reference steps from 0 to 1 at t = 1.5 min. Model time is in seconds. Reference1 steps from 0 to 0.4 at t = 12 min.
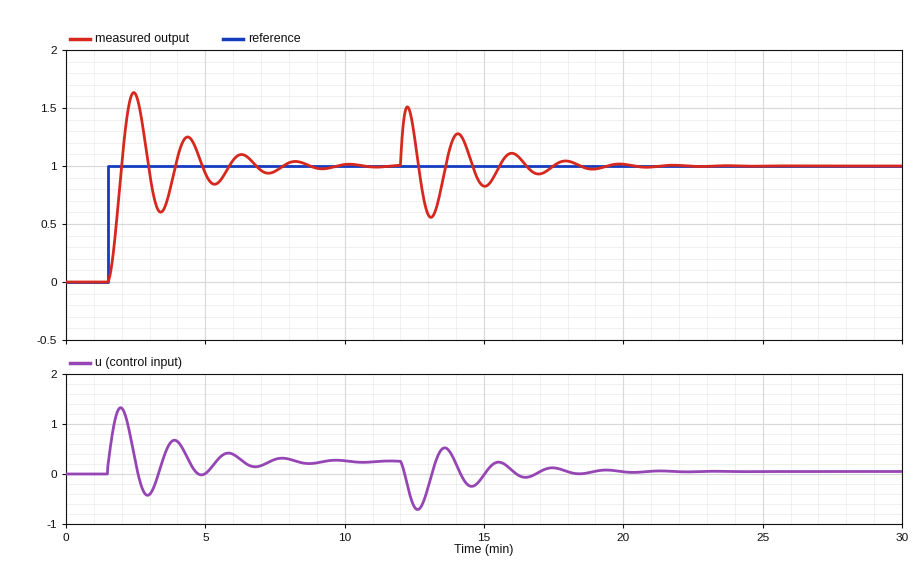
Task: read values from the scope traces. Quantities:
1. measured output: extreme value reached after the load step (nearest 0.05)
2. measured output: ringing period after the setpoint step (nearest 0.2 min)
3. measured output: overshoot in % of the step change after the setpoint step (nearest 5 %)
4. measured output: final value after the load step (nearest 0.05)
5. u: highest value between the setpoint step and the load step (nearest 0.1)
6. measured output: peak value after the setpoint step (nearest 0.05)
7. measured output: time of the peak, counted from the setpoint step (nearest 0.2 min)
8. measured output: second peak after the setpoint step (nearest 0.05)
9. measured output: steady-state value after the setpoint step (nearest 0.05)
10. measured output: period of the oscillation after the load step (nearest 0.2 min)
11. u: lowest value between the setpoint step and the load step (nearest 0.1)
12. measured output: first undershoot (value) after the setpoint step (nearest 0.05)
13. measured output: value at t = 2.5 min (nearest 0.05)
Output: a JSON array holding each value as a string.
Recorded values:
["1.50", "2.0 min", "65 %", "1.00", "1.3", "1.65", "1.0 min", "1.25", "1.00", "1.8 min", "-0.4", "0.60", "1.60"]
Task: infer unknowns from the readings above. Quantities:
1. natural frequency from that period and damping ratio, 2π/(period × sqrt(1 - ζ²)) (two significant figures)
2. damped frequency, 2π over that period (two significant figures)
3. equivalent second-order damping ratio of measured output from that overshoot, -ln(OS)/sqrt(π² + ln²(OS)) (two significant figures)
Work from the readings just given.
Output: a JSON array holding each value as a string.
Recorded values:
["3.2 rad/min", "3.1 rad/min", "0.14"]
